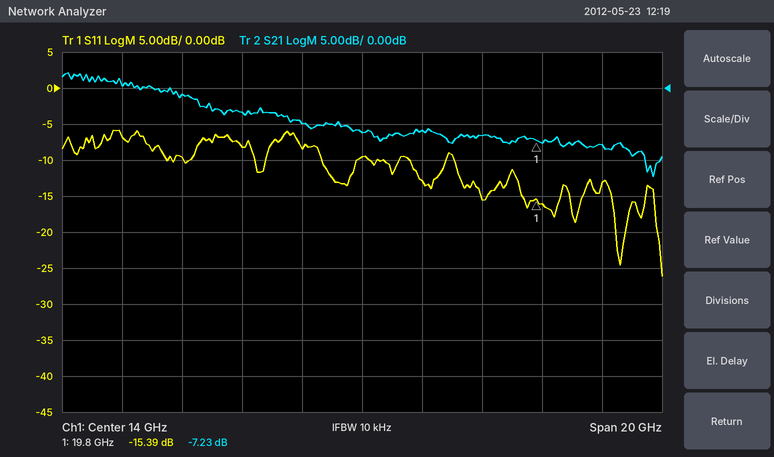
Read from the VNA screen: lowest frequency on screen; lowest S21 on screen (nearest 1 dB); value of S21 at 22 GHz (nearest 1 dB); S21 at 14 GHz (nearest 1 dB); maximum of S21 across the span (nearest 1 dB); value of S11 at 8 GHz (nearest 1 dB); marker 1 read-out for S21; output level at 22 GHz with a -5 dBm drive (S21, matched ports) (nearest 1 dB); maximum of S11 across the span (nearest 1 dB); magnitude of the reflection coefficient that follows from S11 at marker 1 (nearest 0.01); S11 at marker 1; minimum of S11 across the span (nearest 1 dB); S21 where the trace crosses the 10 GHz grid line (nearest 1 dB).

4 GHz
-12 dB
-8 dB
-6 dB
2 dB
-10 dB
-7.23 dB
-13 dBm
-6 dB
0.17
-15.39 dB
-26 dB
-3 dB
